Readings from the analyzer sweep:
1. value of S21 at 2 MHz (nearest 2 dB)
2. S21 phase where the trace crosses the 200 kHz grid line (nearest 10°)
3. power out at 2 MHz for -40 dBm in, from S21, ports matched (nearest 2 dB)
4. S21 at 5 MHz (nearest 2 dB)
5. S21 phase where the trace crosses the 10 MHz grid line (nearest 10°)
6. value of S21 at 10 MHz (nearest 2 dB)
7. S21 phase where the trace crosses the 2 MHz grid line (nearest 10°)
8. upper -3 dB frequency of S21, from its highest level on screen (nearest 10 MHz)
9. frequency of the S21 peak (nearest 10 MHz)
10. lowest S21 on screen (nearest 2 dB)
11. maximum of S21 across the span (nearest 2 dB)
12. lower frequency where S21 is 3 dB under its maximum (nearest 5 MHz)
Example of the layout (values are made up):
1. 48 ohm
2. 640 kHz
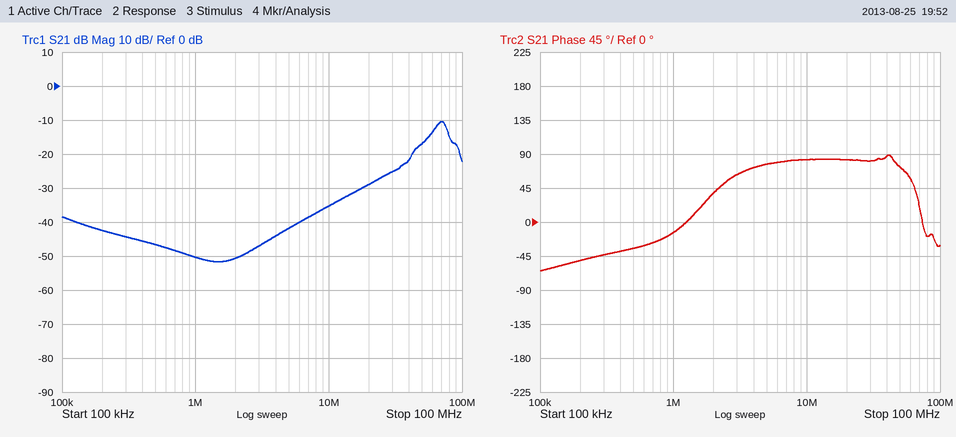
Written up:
1. -50 dB
2. -50°
3. -90 dBm
4. -42 dB
5. 80°
6. -36 dB
7. 40°
8. 80 MHz
9. 70 MHz
10. -52 dB
11. -10 dB
12. 60 MHz
